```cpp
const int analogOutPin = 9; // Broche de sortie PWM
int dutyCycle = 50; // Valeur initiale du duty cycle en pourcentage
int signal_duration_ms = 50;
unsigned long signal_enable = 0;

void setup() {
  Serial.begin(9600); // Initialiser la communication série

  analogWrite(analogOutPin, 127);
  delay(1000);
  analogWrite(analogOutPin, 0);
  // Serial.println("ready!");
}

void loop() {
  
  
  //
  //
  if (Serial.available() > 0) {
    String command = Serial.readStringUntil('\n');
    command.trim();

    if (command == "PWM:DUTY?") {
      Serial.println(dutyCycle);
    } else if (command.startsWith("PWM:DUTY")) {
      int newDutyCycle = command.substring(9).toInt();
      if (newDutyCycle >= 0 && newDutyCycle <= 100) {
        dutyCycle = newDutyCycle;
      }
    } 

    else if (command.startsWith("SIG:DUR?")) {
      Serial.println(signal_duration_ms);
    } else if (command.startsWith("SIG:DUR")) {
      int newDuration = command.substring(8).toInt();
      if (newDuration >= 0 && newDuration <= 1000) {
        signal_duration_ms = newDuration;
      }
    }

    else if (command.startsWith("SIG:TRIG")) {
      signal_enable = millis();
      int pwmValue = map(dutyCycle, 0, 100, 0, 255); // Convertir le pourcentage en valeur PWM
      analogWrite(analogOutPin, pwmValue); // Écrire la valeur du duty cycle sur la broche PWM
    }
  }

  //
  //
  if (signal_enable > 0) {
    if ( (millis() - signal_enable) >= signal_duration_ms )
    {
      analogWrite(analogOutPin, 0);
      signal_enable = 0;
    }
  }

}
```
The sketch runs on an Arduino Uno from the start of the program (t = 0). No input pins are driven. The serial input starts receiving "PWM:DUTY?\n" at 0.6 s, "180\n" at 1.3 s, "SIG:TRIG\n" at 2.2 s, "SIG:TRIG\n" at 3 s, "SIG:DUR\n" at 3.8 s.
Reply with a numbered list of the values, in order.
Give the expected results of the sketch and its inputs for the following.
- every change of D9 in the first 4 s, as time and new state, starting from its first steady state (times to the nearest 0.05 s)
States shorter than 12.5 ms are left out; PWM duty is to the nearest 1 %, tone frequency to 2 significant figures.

1. 0 s PWM 50 %; 1 s low; 2.2 s PWM 50 %; 2.25 s low; 3 s PWM 50 %; 3.05 s low
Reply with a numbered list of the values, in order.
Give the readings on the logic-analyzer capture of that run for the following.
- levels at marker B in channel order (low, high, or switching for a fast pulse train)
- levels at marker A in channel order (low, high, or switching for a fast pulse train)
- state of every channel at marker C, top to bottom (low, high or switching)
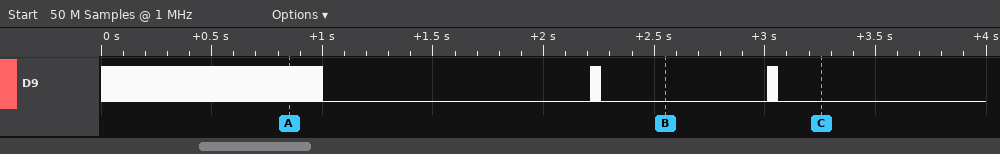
1. D9 low
2. D9 switching
3. D9 low
